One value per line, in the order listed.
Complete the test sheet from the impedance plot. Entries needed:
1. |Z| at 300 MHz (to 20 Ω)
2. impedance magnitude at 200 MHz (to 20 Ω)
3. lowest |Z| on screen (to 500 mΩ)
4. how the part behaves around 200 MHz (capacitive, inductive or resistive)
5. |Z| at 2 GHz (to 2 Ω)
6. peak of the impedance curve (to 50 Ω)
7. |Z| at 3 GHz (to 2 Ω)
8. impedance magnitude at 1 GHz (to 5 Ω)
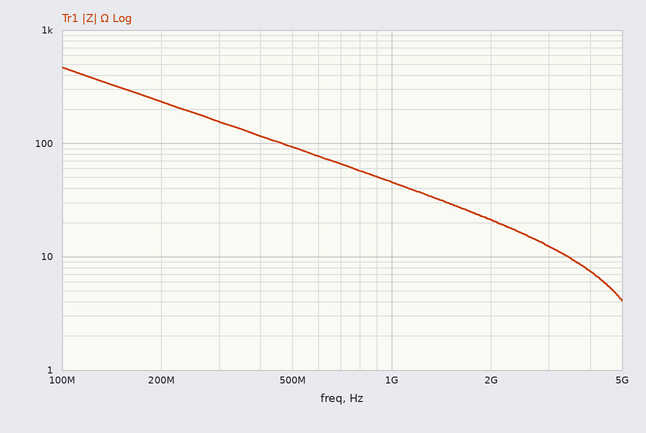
160 Ω
240 Ω
4.0 Ω
capacitive
22 Ω
450 Ω
12 Ω
45 Ω
